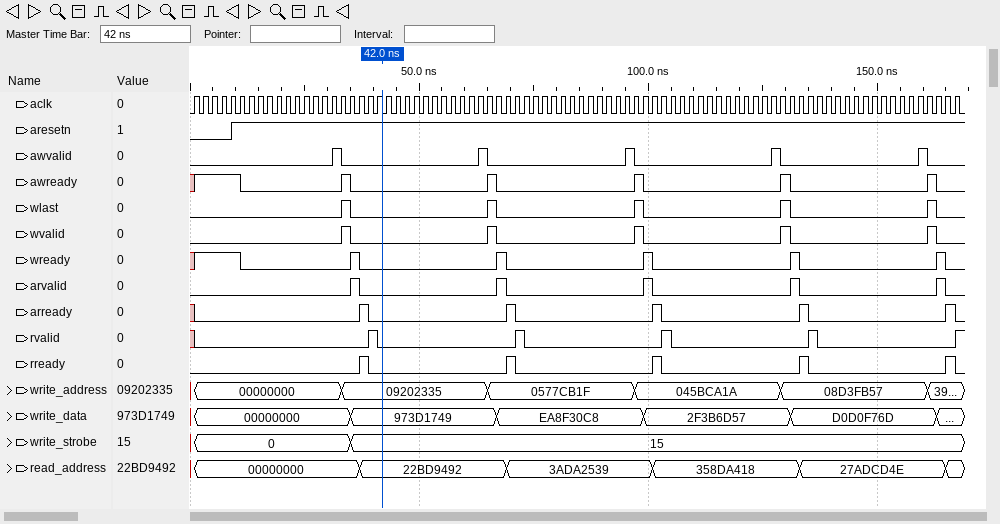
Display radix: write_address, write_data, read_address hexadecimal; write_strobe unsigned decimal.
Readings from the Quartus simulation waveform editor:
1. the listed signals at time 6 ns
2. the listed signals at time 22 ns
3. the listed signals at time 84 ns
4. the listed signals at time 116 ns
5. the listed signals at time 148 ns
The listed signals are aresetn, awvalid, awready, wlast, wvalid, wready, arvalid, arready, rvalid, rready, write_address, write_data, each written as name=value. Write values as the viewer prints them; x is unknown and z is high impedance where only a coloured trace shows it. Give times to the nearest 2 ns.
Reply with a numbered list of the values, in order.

1. aresetn=0, awvalid=0, awready=1, wlast=0, wvalid=0, wready=1, arvalid=0, arready=0, rvalid=0, rready=0, write_address=00000000, write_data=00000000
2. aresetn=1, awvalid=0, awready=0, wlast=0, wvalid=0, wready=0, arvalid=0, arready=0, rvalid=0, rready=0, write_address=00000000, write_data=00000000
3. aresetn=1, awvalid=0, awready=0, wlast=0, wvalid=0, wready=0, arvalid=0, arready=0, rvalid=0, rready=0, write_address=0577CB1F, write_data=EA8F30C8
4. aresetn=1, awvalid=0, awready=0, wlast=0, wvalid=0, wready=0, arvalid=0, arready=0, rvalid=0, rready=0, write_address=045BCA1A, write_data=2F3B6D57
5. aresetn=1, awvalid=0, awready=0, wlast=0, wvalid=0, wready=0, arvalid=0, arready=0, rvalid=0, rready=0, write_address=08D3FB57, write_data=D0D0F76D
